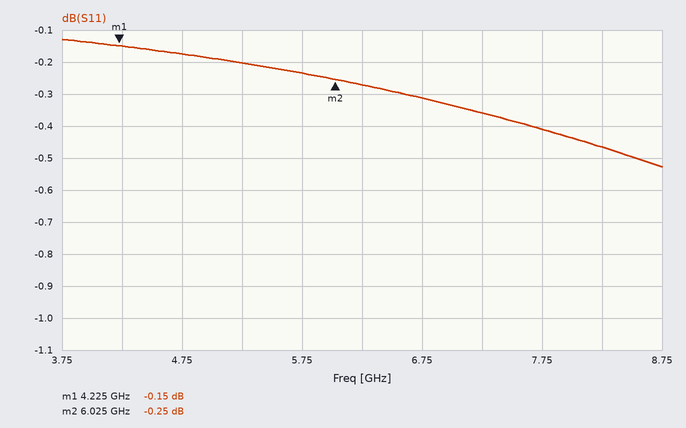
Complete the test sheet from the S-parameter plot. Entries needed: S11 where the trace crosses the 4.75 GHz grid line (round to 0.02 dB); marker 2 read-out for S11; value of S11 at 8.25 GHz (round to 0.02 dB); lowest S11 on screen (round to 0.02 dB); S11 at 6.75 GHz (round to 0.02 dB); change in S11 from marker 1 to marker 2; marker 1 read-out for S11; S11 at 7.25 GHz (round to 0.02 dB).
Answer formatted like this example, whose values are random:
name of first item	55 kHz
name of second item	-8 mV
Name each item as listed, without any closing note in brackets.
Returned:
S11 where the trace crosses the 4.75 GHz grid line	-0.18 dB
marker 2 read-out for S11	-0.25 dB
value of S11 at 8.25 GHz	-0.46 dB
lowest S11 on screen	-0.52 dB
S11 at 6.75 GHz	-0.32 dB
change in S11 from marker 1 to marker 2	-0.10 dB
marker 1 read-out for S11	-0.15 dB
S11 at 7.25 GHz	-0.36 dB
